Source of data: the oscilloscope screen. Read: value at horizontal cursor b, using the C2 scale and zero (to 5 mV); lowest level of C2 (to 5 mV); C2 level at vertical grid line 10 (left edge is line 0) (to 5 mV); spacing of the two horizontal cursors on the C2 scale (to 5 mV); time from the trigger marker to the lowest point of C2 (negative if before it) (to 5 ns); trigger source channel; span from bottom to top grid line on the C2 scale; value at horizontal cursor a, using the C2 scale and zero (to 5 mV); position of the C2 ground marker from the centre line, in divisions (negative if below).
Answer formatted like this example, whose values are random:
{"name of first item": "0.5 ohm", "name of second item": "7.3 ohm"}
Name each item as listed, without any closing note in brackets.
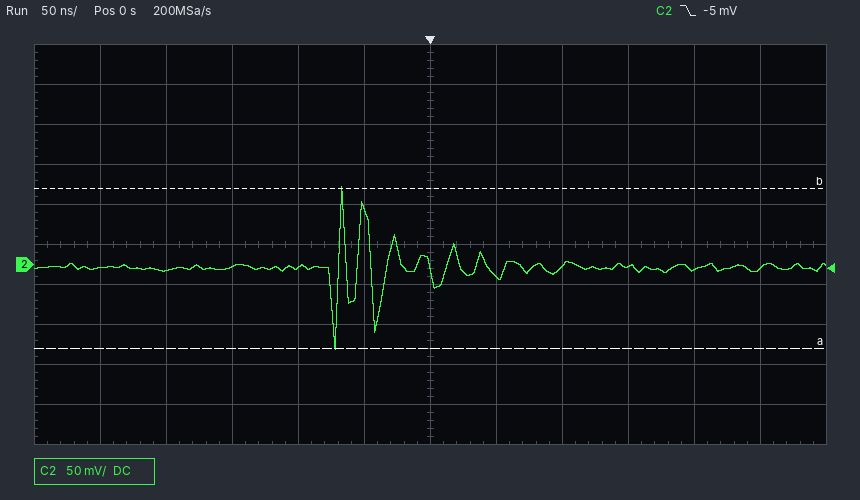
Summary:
{"value at horizontal cursor b, using the C2 scale and zero": "95 mV", "lowest level of C2": "-105 mV", "C2 level at vertical grid line 10 (left edge is line 0)": "-5 mV", "spacing of the two horizontal cursors on the C2 scale": "200 mV", "time from the trigger marker to the lowest point of C2 (negative if before it)": "-70 ns", "trigger source channel": "C2", "span from bottom to top grid line on the C2 scale": "500 mV", "value at horizontal cursor a, using the C2 scale and zero": "-105 mV", "position of the C2 ground marker from the centre line, in divisions": "-0.5 div"}
